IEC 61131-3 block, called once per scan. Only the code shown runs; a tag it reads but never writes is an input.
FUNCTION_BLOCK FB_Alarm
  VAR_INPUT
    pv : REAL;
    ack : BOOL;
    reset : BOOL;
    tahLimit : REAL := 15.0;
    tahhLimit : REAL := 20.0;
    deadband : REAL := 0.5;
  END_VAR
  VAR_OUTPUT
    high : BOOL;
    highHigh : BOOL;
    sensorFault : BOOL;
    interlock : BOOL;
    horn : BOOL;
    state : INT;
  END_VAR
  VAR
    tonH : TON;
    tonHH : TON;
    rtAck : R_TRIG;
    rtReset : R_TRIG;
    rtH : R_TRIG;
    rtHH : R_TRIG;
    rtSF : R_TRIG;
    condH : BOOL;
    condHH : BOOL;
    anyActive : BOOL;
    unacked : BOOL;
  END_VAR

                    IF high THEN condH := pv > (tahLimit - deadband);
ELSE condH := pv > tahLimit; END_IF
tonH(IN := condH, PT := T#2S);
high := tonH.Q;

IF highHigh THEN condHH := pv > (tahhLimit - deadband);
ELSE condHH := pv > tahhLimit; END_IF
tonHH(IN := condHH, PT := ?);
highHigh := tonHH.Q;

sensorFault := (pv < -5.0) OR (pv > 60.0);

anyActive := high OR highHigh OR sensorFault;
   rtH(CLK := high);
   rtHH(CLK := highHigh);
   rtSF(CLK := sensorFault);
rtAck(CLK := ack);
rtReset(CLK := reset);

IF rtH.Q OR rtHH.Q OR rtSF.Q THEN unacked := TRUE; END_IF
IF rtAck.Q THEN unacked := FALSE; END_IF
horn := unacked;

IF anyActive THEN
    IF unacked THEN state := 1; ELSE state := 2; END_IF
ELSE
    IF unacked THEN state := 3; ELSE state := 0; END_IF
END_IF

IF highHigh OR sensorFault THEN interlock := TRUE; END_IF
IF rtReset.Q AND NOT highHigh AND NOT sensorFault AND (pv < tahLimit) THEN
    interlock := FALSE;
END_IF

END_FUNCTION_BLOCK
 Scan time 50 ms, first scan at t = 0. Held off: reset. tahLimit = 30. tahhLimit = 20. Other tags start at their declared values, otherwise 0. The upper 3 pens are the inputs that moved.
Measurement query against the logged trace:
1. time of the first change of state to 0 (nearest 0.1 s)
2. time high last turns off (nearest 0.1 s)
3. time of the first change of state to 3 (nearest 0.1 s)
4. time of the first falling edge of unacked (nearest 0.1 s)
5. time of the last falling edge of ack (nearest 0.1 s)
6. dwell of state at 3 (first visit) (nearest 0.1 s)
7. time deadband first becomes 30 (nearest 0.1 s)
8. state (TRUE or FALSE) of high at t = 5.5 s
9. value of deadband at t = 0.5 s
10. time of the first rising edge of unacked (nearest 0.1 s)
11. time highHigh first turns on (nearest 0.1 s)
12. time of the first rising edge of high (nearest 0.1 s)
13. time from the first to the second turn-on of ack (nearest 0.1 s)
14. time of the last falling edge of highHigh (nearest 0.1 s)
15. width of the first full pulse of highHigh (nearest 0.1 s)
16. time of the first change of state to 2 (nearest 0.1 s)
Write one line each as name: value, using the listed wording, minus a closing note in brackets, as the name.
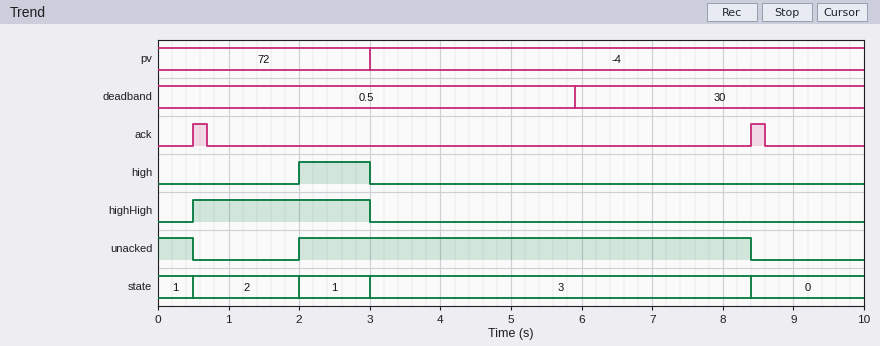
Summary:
time of the first change of state to 0: 8.4 s
time high last turns off: 3.0 s
time of the first change of state to 3: 3.0 s
time of the first falling edge of unacked: 0.5 s
time of the last falling edge of ack: 8.6 s
dwell of state at 3 (first visit): 5.4 s
time deadband first becomes 30: 5.9 s
state (TRUE or FALSE) of high at t = 5.5 s: FALSE
value of deadband at t = 0.5 s: 0.5
time of the first rising edge of unacked: 2.0 s
time highHigh first turns on: 0.5 s
time of the first rising edge of high: 2.0 s
time from the first to the second turn-on of ack: 7.9 s
time of the last falling edge of highHigh: 3.0 s
width of the first full pulse of highHigh: 2.5 s
time of the first change of state to 2: 0.5 s
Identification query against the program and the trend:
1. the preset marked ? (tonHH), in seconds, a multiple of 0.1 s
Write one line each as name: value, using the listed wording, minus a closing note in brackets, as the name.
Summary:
the preset marked ? (tonHH), in seconds, a multiple of 0.1 s: 0.5 s
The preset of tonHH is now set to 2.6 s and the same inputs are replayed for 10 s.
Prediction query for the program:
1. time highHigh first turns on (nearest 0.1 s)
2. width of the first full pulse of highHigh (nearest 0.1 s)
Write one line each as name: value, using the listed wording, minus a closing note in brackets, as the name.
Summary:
time highHigh first turns on: 2.6 s
width of the first full pulse of highHigh: 0.4 s
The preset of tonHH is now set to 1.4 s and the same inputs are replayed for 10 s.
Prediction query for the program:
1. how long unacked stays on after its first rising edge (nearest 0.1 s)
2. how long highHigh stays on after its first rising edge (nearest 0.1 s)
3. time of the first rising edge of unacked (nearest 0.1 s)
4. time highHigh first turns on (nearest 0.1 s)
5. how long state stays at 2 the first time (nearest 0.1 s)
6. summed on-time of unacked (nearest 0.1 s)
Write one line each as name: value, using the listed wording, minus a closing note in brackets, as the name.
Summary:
how long unacked stays on after its first rising edge: 7.0 s
how long highHigh stays on after its first rising edge: 1.6 s
time of the first rising edge of unacked: 1.4 s
time highHigh first turns on: 1.4 s
how long state stays at 2 the first time: 0.9 s
summed on-time of unacked: 7.5 s
